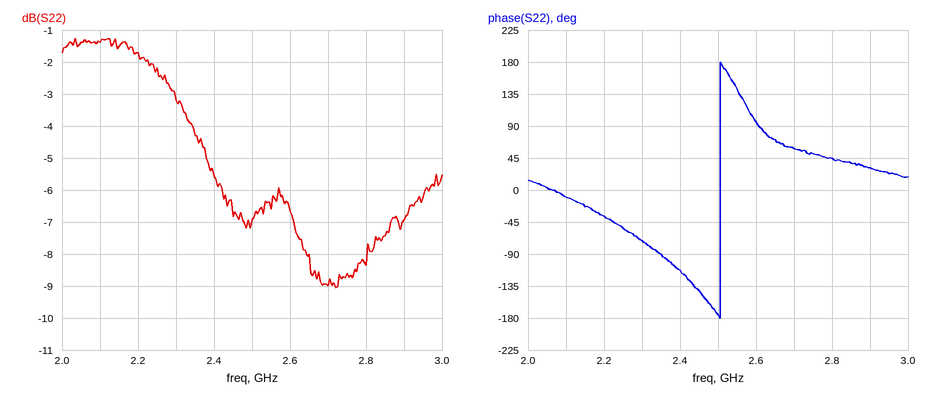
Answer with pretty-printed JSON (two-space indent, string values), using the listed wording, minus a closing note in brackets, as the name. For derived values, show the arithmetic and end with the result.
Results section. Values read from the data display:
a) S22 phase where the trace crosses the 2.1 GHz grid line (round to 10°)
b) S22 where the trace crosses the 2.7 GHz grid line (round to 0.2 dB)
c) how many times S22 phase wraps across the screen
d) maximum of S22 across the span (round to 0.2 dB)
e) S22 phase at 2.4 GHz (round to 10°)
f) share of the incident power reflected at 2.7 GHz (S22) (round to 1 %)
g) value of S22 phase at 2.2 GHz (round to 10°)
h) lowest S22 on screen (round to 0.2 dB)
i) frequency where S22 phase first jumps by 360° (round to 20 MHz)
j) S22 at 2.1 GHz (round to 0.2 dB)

{
  "S22 phase where the trace crosses the 2.1 GHz grid line": "-10°",
  "S22 where the trace crosses the 2.7 GHz grid line": "-9.0 dB",
  "how many times S22 phase wraps across the screen": "1",
  "maximum of S22 across the span": "-1.2 dB",
  "S22 phase at 2.4 GHz": "-110°",
  "share of the incident power reflected at 2.7 GHz (S22)": "10^(-9/10) ≈ 13 %",
  "value of S22 phase at 2.2 GHz": "-40°",
  "lowest S22 on screen": "-9.0 dB",
  "frequency where S22 phase first jumps by 360°": "2.50 GHz",
  "S22 at 2.1 GHz": "-1.4 dB"
}
